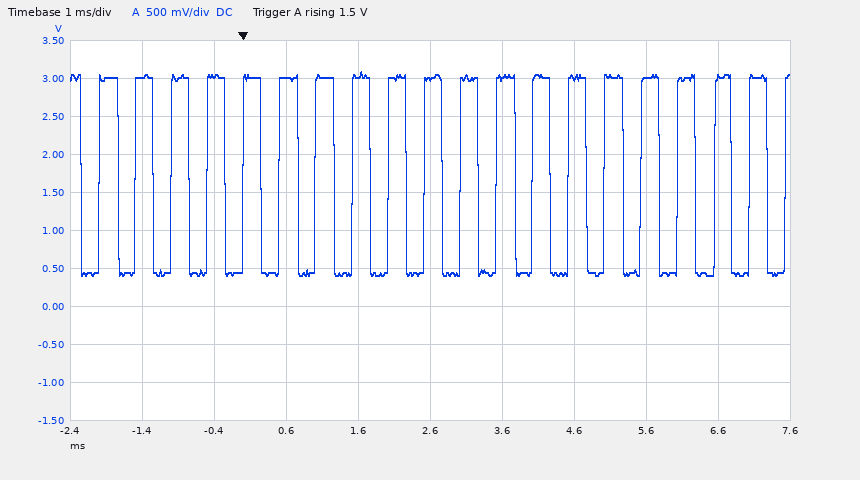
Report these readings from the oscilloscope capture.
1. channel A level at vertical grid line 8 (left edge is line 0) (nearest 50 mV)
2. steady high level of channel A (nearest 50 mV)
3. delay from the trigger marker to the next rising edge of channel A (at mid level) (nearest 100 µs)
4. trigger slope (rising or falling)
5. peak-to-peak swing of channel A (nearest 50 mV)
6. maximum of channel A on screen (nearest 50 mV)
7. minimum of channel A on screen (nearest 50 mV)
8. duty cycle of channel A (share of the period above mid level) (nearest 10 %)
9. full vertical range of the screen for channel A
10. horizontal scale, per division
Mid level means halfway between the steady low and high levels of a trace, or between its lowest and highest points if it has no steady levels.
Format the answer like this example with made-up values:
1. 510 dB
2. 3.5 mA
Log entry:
1. 3.00 V
2. 3.00 V
3. 500 µs
4. rising
5. 2.70 V
6. 3.10 V
7. 400 mV
8. 50 %
9. 5 V
10. 1 ms
